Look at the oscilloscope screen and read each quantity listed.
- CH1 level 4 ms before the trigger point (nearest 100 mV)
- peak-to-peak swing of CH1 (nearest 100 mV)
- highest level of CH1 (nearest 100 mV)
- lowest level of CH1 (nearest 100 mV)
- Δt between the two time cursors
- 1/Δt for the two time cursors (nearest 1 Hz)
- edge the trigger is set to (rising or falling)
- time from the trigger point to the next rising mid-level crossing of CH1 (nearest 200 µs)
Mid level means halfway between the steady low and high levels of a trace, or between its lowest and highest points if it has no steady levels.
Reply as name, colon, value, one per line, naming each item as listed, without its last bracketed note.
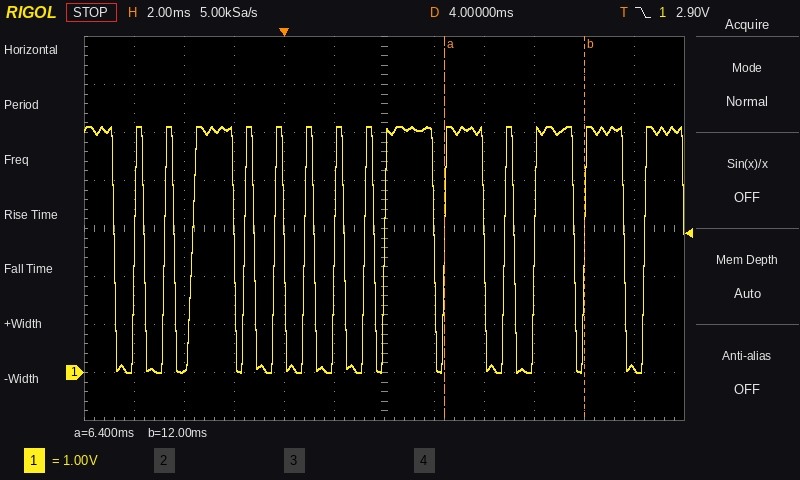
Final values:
CH1 level 4 ms before the trigger point: 100 mV
peak-to-peak swing of CH1: 5.1 V
highest level of CH1: 5.1 V
lowest level of CH1: 0.0 V
Δt between the two time cursors: 5.6 ms
1/Δt for the two time cursors: 179 Hz
edge the trigger is set to: falling
time from the trigger point to the next rising mid-level crossing of CH1: 800 µs
